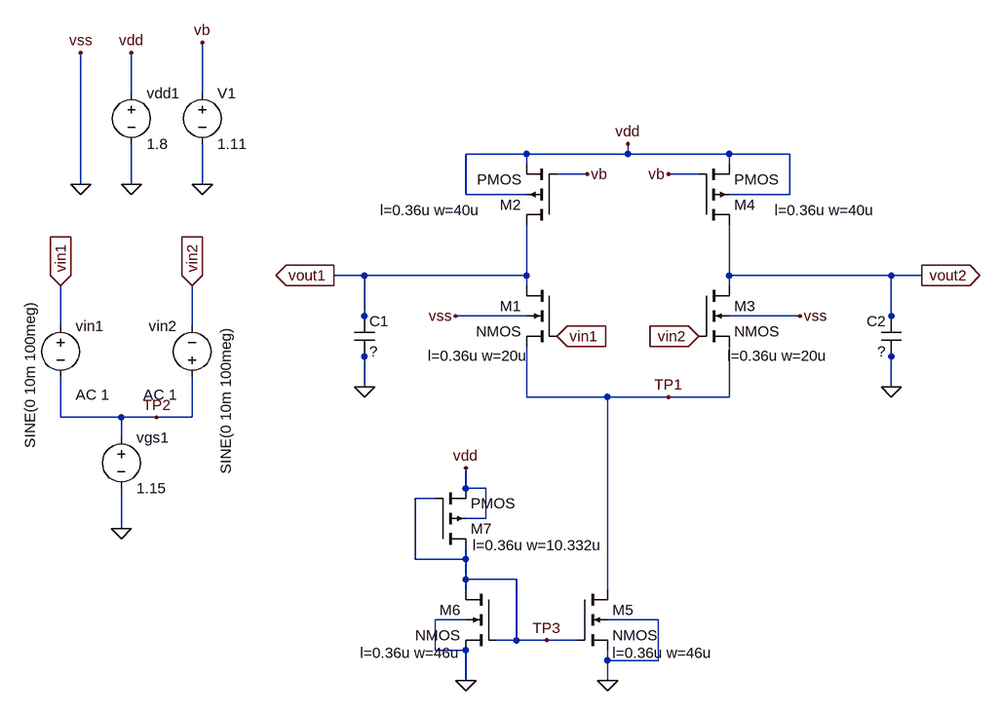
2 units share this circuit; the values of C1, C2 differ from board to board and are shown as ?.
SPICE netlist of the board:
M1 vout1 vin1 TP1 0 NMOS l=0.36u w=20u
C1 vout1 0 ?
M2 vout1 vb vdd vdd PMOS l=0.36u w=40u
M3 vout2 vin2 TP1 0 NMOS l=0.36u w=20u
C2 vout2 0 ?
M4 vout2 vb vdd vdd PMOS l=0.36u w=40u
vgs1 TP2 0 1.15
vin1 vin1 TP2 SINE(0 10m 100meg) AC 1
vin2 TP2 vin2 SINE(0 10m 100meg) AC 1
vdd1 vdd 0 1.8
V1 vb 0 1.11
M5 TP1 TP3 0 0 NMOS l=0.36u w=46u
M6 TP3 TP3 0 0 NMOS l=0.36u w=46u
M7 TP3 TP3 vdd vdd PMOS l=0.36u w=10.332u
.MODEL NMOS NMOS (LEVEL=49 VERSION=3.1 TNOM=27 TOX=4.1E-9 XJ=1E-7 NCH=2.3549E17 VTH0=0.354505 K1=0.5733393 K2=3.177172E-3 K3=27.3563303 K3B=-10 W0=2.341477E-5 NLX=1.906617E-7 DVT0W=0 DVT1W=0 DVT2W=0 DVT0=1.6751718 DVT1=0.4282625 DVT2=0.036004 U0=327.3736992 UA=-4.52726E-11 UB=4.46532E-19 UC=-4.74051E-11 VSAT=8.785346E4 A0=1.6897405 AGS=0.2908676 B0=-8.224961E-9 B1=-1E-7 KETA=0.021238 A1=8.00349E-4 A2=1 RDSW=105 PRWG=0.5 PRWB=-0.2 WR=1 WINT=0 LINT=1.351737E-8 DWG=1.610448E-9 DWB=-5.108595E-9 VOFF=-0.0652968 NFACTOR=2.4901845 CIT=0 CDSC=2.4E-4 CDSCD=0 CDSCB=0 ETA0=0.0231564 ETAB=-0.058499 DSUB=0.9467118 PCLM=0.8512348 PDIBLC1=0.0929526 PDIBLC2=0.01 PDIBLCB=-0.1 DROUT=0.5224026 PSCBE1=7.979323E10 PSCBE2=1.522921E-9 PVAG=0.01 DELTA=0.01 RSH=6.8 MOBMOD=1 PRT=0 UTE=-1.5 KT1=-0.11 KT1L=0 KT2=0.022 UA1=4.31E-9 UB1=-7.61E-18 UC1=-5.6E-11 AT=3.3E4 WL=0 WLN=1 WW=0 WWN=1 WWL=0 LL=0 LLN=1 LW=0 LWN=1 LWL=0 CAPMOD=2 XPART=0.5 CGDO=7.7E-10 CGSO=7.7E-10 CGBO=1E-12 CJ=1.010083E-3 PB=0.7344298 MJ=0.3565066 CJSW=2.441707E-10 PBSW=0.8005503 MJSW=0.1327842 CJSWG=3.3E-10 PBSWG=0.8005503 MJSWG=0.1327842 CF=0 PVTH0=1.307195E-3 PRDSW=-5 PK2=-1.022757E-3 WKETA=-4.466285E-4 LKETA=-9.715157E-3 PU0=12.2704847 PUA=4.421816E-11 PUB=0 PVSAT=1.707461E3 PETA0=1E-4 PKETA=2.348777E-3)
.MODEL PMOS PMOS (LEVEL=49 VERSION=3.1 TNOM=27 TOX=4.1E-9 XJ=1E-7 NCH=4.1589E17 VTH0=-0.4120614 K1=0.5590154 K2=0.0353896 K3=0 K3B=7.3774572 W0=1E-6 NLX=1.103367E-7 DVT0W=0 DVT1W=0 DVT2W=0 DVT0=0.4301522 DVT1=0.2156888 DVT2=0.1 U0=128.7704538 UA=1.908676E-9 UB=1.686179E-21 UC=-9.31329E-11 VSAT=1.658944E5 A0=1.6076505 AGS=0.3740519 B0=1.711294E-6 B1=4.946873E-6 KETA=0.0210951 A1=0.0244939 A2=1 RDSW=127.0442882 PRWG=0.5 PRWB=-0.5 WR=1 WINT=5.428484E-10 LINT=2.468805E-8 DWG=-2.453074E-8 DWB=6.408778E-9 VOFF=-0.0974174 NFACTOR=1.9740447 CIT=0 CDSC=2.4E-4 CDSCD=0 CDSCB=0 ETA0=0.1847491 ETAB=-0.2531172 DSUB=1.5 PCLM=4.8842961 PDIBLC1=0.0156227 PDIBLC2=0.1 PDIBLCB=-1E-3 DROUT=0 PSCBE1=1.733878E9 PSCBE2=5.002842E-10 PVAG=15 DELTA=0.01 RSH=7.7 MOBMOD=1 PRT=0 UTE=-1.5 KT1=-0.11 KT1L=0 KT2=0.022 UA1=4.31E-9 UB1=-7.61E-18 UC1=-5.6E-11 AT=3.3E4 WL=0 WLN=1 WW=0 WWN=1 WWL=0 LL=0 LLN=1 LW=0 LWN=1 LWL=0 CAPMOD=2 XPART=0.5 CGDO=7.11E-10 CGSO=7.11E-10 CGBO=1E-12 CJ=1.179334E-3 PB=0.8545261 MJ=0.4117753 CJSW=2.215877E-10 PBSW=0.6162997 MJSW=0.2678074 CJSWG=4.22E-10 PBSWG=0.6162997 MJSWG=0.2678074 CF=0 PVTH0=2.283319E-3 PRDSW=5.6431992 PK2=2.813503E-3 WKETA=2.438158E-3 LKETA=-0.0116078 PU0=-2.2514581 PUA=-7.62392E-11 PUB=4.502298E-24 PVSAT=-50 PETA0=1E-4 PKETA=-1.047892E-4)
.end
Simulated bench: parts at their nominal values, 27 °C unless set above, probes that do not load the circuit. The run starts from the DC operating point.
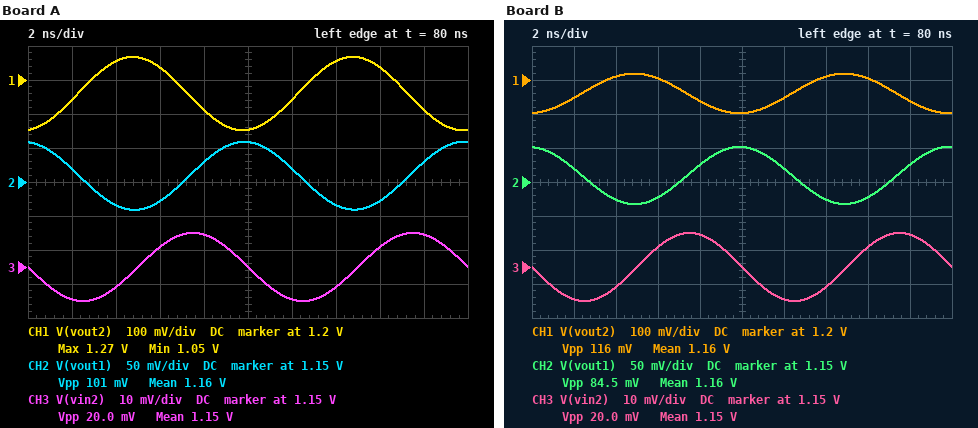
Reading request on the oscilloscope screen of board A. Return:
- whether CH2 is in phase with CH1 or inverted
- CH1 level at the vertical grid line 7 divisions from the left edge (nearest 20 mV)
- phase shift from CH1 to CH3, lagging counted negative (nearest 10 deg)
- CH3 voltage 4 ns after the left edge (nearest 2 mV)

inverted
1.26 V
-100 deg
1.144 V
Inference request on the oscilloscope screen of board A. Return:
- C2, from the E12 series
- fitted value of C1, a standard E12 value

270 fF
680 fF
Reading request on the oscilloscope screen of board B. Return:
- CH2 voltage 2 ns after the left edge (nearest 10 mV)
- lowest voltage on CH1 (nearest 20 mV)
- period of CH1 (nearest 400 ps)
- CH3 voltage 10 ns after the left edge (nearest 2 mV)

1.17 V
1.10 V
10.0 ns
1.150 V
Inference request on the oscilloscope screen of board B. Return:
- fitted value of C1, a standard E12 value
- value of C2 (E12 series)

820 fF
560 fF
